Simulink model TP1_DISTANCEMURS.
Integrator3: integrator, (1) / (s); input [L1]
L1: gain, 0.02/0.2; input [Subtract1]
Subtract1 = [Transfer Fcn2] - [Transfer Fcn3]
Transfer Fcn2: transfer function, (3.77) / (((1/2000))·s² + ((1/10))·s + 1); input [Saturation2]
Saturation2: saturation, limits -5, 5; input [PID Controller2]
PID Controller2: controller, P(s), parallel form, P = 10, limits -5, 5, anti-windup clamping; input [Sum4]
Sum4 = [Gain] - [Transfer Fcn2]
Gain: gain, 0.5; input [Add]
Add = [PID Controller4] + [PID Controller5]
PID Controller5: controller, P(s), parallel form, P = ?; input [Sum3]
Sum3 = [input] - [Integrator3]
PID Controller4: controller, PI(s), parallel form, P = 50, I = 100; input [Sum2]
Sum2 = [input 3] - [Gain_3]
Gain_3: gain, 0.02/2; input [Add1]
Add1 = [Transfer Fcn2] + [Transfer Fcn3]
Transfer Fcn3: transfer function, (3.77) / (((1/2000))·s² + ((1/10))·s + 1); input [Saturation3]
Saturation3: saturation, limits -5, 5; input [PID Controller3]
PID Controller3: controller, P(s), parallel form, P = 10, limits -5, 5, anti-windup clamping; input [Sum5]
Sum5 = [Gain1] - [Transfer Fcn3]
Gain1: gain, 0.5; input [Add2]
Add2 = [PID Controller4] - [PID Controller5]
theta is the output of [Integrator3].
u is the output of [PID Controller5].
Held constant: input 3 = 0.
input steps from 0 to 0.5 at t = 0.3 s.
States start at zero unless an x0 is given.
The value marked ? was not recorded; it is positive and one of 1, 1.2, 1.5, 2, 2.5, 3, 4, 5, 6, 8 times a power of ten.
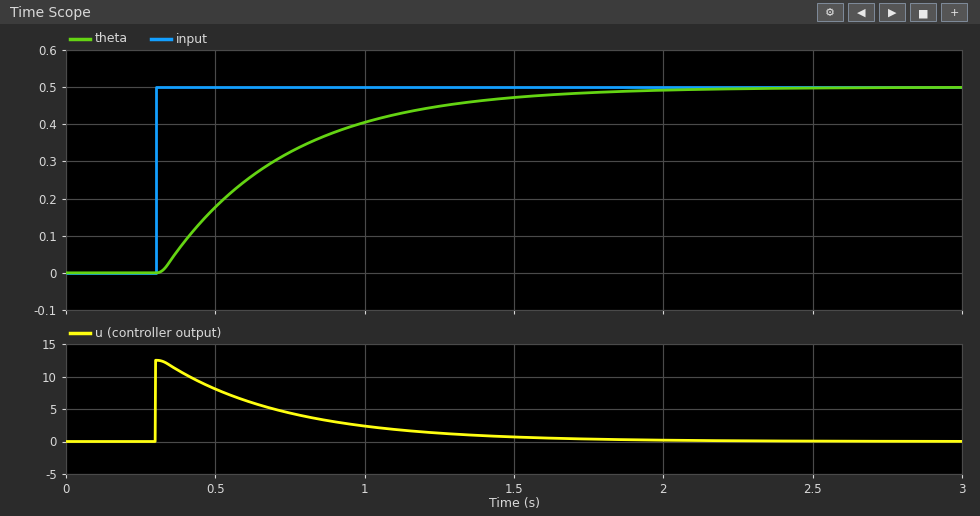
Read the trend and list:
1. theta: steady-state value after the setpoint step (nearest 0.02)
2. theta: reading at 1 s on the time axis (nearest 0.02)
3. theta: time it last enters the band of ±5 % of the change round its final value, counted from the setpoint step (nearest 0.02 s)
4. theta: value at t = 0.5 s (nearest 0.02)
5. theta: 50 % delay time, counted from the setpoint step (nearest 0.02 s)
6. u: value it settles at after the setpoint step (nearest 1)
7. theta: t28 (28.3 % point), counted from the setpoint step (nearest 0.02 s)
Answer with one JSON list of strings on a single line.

["0.50", "0.40", "1.24 s", "0.18", "0.30 s", "0", "0.16 s"]
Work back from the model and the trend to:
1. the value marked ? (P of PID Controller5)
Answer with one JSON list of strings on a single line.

["25"]
